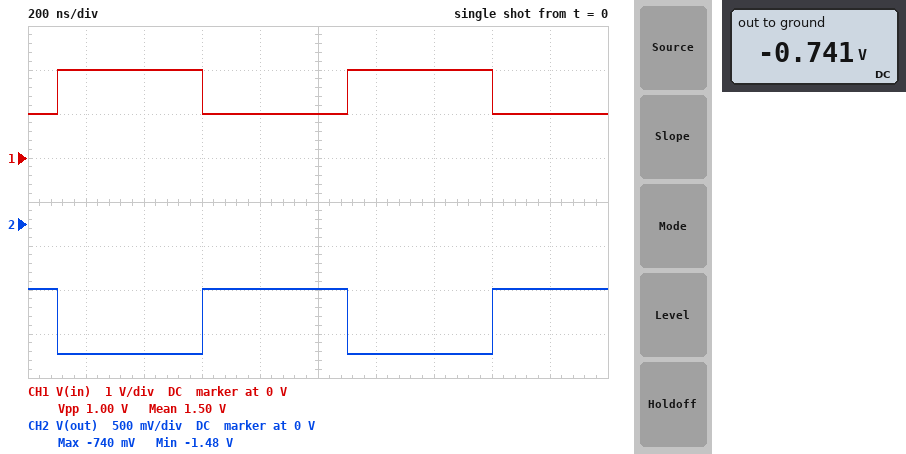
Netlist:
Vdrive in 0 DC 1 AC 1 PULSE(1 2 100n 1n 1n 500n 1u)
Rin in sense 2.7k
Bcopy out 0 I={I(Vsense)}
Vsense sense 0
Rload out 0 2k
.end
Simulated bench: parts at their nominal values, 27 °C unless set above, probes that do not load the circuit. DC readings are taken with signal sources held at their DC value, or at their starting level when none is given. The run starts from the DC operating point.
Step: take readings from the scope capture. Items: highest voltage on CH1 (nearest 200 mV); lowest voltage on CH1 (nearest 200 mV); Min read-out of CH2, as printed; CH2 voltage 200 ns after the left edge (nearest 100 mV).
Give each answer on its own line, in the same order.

2.0 V
1.0 V
-1.48 V
-1.5 V
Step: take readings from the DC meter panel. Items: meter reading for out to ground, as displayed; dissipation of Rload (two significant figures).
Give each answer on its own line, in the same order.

-0.741 V
270 µW
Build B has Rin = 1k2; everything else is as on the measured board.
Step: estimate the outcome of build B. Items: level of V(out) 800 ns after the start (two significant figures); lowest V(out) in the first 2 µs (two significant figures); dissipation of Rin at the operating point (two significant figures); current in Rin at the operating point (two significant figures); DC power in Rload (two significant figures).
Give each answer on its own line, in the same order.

-1.7 V
-3.3 V
830 µW
830 µA
1.4 mW
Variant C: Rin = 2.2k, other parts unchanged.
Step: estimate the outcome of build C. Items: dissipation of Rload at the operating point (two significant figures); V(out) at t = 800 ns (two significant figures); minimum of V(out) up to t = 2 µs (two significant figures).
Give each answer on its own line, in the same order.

410 µW
-910 mV
-1.8 V
